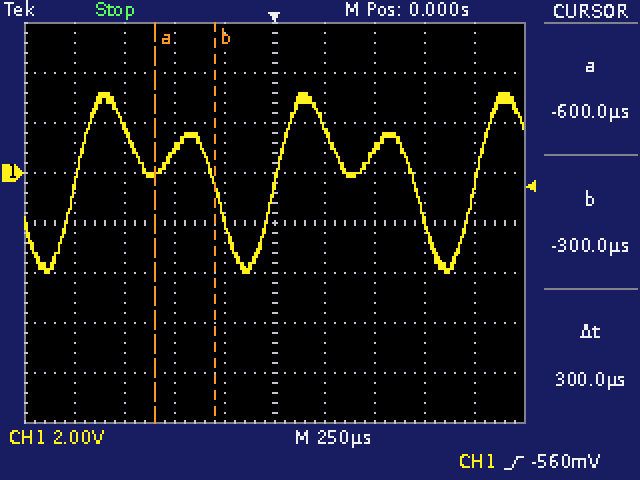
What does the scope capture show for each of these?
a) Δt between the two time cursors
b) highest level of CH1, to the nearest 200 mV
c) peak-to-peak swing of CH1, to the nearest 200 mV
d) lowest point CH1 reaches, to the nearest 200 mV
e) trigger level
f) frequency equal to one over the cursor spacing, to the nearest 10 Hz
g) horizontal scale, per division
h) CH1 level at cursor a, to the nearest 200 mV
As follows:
300 µs
3.2 V
7.2 V
-4.0 V
-560 mV
3.33 kHz
250 µs
0.0 V
